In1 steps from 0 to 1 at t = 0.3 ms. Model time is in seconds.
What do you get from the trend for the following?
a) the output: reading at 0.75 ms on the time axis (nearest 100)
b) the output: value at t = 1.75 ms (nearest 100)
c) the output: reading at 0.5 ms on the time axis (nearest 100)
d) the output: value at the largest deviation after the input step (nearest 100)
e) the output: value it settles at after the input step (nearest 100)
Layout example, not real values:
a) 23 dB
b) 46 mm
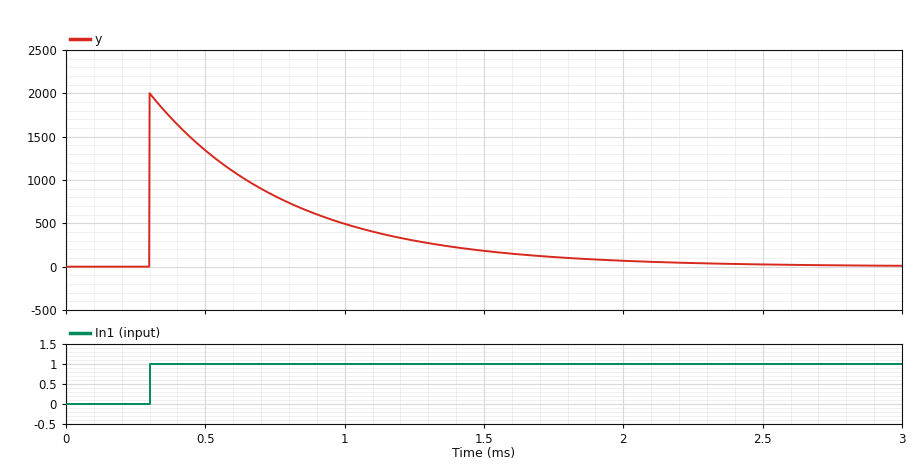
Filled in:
a) 800
b) 100
c) 1300
d) 2000
e) 0
